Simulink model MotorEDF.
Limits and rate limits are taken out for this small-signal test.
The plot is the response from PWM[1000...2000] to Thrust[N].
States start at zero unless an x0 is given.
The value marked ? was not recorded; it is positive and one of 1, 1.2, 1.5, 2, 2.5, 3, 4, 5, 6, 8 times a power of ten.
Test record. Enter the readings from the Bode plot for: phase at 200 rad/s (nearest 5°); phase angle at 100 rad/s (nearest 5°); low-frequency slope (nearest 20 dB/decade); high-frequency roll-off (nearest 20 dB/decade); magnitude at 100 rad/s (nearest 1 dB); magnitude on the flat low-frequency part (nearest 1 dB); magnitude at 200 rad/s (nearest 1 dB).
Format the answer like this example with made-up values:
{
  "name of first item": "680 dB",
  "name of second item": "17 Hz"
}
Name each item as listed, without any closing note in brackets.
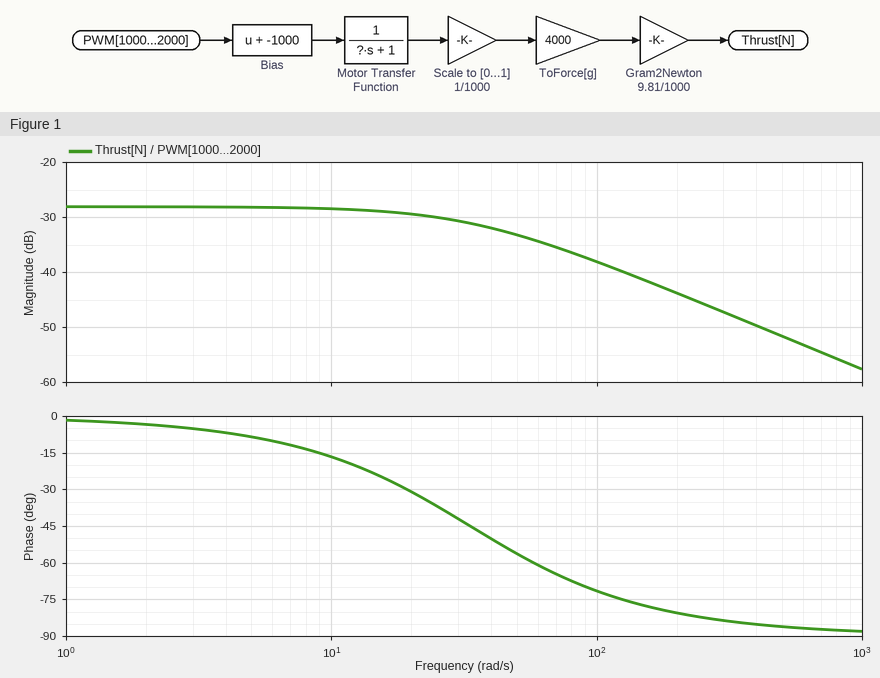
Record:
{
  "phase at 200 rad/s": "-80°",
  "phase angle at 100 rad/s": "-70°",
  "low-frequency slope": "0 dB/decade",
  "high-frequency roll-off": "-20 dB/decade",
  "magnitude at 100 rad/s": "-38 dB",
  "magnitude on the flat low-frequency part": "-28 dB",
  "magnitude at 200 rad/s": "-44 dB"
}
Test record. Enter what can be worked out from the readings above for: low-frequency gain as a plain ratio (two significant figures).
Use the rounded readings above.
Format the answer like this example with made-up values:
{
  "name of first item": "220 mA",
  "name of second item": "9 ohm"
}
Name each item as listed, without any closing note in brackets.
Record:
{
  "low-frequency gain as a plain ratio": "0.040"
}
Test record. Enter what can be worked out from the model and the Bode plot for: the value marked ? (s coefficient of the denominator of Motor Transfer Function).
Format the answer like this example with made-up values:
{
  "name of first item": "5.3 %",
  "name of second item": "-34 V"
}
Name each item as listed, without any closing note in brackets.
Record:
{
  "the value marked ?": "0.03"
}
